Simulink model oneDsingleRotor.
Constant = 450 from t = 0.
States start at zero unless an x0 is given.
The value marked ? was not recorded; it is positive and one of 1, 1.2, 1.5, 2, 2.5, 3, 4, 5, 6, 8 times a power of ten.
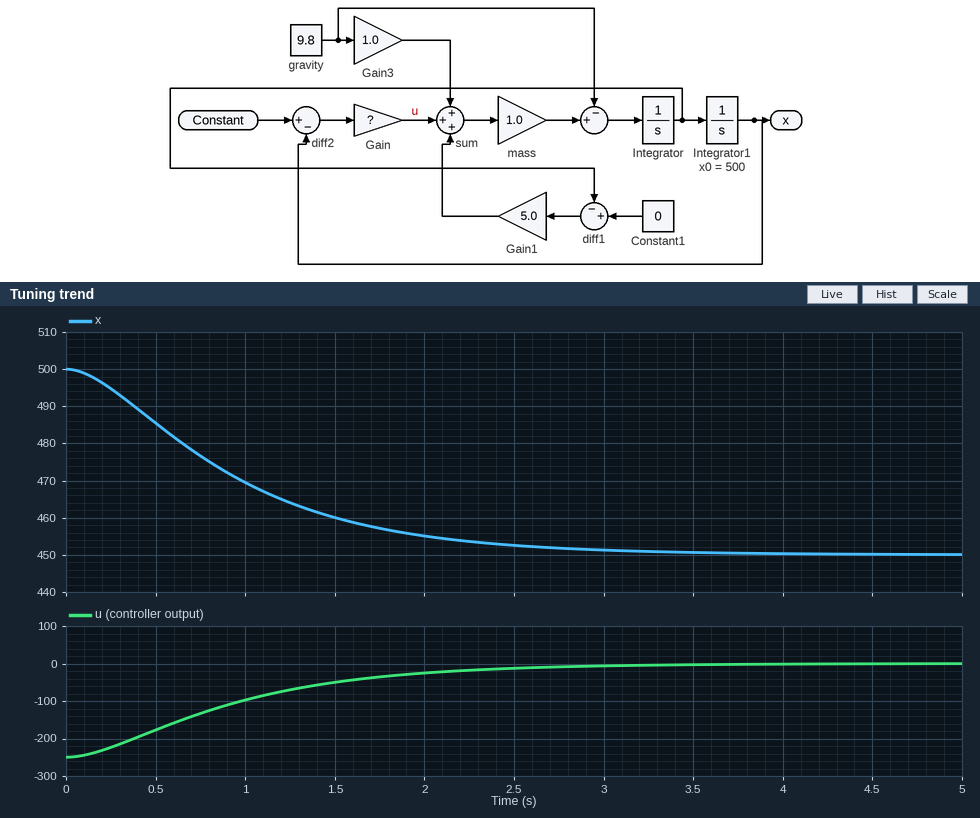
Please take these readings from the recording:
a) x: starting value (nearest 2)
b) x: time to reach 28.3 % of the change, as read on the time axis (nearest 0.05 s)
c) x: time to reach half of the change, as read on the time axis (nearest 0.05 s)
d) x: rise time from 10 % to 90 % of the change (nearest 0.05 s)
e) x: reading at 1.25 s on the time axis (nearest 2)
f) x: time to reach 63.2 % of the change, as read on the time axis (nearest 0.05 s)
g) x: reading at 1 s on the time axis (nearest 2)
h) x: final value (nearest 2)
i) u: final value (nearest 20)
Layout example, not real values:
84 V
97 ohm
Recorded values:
500
0.50 s
0.80 s
1.75 s
464
1.05 s
470
450
0
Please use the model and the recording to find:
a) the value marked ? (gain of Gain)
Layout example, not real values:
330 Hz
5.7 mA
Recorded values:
5
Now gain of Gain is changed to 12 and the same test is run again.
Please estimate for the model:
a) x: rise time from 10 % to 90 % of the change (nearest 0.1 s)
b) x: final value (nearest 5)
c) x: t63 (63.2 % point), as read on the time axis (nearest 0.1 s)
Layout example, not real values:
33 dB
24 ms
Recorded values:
0.6 s
450
0.5 s
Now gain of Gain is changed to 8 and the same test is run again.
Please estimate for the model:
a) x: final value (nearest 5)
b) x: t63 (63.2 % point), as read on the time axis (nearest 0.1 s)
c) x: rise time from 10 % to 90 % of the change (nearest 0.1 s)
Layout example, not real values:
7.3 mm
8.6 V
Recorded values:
450
0.7 s
1.0 s
